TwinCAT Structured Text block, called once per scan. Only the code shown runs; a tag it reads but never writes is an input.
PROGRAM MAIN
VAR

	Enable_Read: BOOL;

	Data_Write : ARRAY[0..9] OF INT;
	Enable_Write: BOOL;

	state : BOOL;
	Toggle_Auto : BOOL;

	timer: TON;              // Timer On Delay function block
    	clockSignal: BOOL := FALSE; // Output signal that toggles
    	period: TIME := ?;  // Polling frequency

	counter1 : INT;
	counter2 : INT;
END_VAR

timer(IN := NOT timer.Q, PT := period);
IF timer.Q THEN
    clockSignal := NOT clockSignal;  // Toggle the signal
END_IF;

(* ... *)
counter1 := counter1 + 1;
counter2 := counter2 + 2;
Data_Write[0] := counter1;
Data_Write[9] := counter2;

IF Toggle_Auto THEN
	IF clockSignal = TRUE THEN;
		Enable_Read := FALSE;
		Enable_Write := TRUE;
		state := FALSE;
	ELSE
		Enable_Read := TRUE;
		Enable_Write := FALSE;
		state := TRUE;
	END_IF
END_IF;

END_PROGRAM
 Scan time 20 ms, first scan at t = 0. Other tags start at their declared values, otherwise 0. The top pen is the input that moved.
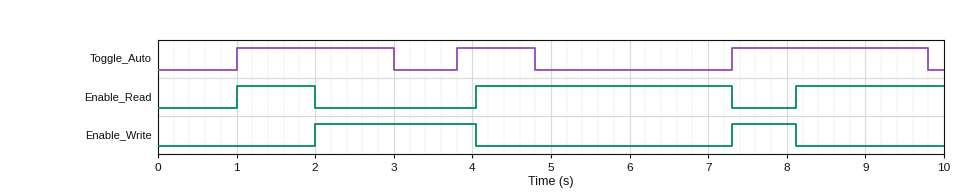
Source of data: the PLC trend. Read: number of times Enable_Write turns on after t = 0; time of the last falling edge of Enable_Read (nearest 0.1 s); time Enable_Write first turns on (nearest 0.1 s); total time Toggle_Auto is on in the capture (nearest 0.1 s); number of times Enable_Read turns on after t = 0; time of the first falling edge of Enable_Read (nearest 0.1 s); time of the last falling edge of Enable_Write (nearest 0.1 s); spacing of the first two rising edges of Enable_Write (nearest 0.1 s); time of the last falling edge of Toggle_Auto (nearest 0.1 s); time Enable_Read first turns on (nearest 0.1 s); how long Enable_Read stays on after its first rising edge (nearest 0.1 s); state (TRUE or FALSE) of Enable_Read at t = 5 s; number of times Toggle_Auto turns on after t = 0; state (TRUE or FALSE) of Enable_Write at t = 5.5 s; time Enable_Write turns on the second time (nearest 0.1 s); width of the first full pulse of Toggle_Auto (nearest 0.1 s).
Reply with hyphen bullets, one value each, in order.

- 2
- 7.3 s
- 2.0 s
- 5.5 s
- 3
- 2.0 s
- 8.1 s
- 5.3 s
- 9.8 s
- 1.0 s
- 1.0 s
- TRUE
- 3
- FALSE
- 7.3 s
- 2.0 s
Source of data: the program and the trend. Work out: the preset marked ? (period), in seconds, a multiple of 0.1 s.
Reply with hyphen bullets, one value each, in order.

- 2.0 s
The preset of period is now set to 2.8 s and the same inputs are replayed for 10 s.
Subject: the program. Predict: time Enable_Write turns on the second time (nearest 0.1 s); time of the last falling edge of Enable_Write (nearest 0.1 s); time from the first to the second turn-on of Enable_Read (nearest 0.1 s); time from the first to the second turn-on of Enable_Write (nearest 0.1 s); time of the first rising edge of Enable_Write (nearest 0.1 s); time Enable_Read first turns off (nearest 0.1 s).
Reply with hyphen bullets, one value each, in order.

- 8.5 s
- 7.3 s
- 6.3 s
- 5.7 s
- 2.8 s
- 2.8 s
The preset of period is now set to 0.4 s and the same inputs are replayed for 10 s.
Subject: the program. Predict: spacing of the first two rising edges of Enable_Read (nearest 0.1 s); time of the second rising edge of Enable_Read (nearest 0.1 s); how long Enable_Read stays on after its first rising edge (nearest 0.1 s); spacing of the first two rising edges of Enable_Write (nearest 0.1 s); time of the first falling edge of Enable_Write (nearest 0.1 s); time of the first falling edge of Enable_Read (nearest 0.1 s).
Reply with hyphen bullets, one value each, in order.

- 0.7 s
- 1.7 s
- 0.3 s
- 0.9 s
- 1.7 s
- 1.3 s
